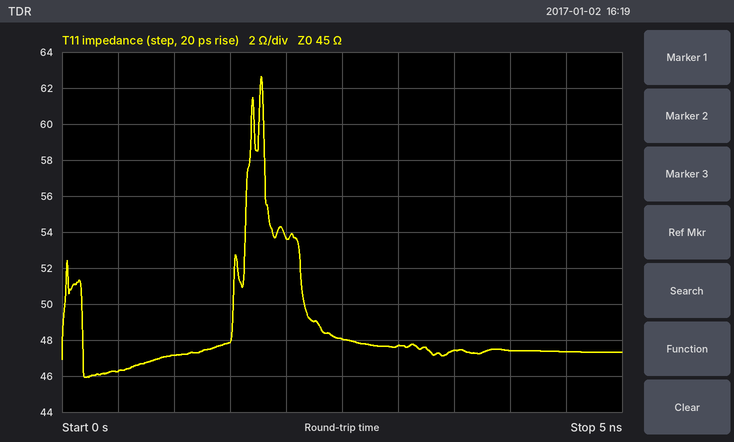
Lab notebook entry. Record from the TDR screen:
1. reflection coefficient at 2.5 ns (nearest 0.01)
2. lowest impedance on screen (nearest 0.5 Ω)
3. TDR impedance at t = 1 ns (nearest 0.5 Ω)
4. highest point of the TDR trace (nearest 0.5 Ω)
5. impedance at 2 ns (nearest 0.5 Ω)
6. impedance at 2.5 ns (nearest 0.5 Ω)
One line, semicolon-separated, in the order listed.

+0.03; 46.0 Ω; 47.0 Ω; 62.5 Ω; 53.5 Ω; 48.0 Ω
